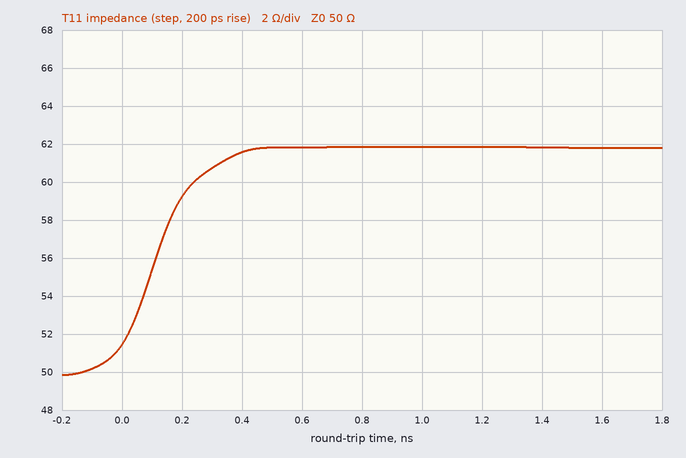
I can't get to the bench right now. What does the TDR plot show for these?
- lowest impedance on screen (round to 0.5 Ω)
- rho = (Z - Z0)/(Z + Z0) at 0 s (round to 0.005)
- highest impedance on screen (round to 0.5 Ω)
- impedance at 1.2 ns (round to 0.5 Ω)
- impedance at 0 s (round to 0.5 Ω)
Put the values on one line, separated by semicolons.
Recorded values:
50.0 Ω; +0.015; 62.0 Ω; 62.0 Ω; 51.5 Ω
